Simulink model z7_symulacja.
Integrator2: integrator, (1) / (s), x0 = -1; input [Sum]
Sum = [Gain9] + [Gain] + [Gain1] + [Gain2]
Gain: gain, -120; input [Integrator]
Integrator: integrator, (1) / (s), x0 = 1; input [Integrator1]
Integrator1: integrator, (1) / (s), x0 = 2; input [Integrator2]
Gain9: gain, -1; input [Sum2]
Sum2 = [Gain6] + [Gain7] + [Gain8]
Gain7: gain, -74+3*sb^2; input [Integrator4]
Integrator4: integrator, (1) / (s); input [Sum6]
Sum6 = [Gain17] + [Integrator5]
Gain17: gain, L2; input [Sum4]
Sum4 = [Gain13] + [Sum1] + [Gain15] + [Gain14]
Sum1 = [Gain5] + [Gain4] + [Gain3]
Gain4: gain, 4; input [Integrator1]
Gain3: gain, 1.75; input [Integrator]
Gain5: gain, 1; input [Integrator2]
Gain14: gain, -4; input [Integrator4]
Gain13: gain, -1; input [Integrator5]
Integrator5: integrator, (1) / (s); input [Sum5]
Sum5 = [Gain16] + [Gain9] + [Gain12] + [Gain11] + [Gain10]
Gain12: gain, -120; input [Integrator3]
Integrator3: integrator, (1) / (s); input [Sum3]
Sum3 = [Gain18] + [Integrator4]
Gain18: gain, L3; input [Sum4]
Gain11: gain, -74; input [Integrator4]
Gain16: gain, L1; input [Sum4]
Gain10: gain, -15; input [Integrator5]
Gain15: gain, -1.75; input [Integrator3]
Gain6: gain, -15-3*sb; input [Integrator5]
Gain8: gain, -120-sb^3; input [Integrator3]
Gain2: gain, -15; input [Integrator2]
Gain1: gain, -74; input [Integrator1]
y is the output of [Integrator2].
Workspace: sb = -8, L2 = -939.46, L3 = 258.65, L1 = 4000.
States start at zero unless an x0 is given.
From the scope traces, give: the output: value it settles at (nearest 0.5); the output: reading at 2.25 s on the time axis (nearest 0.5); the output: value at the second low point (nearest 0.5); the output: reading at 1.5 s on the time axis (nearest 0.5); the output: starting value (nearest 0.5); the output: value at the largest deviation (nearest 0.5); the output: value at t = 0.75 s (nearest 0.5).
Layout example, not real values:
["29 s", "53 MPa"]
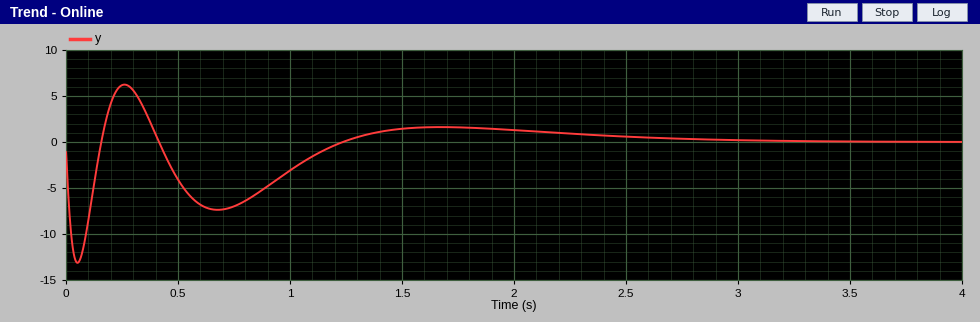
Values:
["0.0", "1.0", "-7.5", "1.5", "-1.0", "-13.0", "-7.0"]
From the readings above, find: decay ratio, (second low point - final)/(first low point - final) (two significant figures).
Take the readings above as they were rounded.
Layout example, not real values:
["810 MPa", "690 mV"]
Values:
["0.58"]
